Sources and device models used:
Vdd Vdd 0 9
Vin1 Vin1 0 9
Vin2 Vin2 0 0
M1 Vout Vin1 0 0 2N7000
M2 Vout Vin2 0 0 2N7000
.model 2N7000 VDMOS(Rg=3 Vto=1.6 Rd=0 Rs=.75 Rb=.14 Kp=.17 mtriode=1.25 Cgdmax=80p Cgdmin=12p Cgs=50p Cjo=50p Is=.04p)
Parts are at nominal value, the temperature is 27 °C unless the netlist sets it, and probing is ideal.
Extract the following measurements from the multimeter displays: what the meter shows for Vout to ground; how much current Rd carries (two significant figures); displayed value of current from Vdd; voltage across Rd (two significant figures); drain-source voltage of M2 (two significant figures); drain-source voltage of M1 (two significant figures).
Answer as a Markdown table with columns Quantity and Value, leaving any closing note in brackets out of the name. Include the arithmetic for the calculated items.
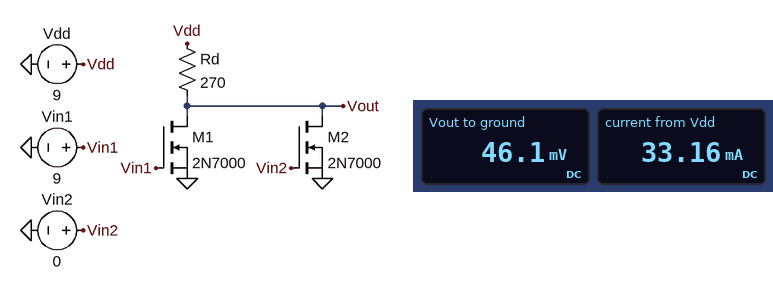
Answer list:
| Quantity | Value |
|---|---|
| what the meter shows for Vout to ground | 46.1 mV |
| how much current Rd carries | (9 V - 46.1 mV) / 270 Ω = 33 mA |
| displayed value of current from Vdd | 33.16 mA |
| voltage across Rd | 9 V - 46.1 mV = 9.0 V |
| drain-source voltage of M2 | 46.1 mV = 46 mV |
| drain-source voltage of M1 | 46.1 mV = 46 mV |
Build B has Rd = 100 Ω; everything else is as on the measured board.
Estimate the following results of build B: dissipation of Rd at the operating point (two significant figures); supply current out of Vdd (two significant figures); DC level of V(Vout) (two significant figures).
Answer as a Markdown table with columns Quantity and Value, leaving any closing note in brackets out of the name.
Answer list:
| Quantity | Value |
|---|---|
| dissipation of Rd at the operating point | 790 mW |
| supply current out of Vdd | 89 mA |
| DC level of V(Vout) | 120 mV |
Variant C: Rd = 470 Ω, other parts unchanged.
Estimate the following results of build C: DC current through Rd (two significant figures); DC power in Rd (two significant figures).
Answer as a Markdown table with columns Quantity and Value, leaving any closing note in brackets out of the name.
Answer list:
| Quantity | Value |
|---|---|
| DC current through Rd | 19 mA |
| DC power in Rd | 170 mW |
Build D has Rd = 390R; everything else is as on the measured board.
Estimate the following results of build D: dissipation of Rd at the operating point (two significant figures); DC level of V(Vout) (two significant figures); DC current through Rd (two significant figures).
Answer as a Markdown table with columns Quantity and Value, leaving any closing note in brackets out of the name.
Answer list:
| Quantity | Value |
|---|---|
| dissipation of Rd at the operating point | 210 mW |
| DC level of V(Vout) | 32 mV |
| DC current through Rd | 23 mA |
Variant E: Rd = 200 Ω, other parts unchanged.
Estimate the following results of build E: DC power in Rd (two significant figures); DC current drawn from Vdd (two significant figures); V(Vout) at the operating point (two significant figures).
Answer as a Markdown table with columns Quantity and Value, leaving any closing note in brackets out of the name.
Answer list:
| Quantity | Value |
|---|---|
| DC power in Rd | 400 mW |
| DC current drawn from Vdd | 45 mA |
| V(Vout) at the operating point | 62 mV |
